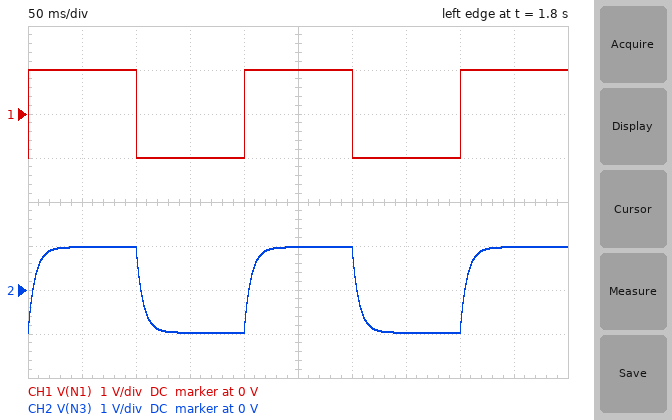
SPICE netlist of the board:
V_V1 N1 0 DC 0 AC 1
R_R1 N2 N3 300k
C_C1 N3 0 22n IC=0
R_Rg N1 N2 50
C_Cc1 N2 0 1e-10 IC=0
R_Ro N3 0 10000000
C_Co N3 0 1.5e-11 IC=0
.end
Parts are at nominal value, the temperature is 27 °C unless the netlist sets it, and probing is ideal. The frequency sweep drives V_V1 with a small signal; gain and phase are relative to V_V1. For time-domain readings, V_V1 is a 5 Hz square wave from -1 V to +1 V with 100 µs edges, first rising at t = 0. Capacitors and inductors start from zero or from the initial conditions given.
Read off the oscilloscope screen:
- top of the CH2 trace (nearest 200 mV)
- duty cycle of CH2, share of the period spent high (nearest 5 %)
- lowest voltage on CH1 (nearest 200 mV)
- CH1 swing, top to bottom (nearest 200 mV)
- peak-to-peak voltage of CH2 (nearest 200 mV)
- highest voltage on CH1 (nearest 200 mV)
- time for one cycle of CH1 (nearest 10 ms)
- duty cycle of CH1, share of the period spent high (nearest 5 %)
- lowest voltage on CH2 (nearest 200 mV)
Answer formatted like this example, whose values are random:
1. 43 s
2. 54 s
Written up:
1. 1.0 V
2. 50 %
3. -1.0 V
4. 2.0 V
5. 2.0 V
6. 1.0 V
7. 200 ms
8. 50 %
9. -1.0 V
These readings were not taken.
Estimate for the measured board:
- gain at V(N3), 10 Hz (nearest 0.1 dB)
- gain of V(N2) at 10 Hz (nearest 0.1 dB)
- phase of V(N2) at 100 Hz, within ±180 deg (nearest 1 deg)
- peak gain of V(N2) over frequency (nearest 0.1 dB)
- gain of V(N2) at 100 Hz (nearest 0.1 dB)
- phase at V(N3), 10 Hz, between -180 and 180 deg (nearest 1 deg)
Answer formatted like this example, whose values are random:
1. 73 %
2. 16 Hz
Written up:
1. -0.9 dB
2. 0 dB
3. 0 deg
4. 0 dB
5. 0 dB
6. -22 deg
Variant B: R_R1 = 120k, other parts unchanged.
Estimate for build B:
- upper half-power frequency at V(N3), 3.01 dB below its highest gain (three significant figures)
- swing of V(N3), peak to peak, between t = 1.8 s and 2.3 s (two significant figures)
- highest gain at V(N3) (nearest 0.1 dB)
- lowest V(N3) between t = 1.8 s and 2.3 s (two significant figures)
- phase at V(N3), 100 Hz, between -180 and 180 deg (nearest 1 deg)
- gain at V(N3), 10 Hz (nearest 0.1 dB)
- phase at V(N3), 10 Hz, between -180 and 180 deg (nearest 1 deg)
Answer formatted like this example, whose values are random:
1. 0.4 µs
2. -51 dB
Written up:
1. 60.9 Hz
2. 2.0 V
3. -0.1 dB
4. -990 mV
5. -59 deg
6. -0.2 dB
7. -9 deg
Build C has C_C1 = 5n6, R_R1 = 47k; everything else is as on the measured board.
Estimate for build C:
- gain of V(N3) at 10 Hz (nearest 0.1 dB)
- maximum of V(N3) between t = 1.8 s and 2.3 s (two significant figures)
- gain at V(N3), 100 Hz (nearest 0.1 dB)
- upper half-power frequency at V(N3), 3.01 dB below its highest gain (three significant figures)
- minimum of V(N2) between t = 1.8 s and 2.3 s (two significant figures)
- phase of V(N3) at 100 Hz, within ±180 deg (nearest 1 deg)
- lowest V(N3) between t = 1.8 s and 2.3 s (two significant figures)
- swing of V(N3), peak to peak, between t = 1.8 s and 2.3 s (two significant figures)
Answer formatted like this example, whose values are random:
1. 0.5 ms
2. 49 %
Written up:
1. 0 dB
2. 1.0 V
3. -0.2 dB
4. 605 Hz
5. -1.0 V
6. -9 deg
7. -1.0 V
8. 2.0 V
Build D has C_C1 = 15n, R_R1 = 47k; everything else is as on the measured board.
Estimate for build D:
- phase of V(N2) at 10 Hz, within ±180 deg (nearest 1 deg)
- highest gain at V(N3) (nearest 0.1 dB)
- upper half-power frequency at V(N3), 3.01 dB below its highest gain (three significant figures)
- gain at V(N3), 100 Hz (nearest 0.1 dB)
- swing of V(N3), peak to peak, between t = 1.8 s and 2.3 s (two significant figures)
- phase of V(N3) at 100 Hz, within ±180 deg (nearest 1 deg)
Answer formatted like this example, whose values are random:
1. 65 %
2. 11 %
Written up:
1. 0 deg
2. 0 dB
3. 226 Hz
4. -0.8 dB
5. 2.0 V
6. -24 deg
